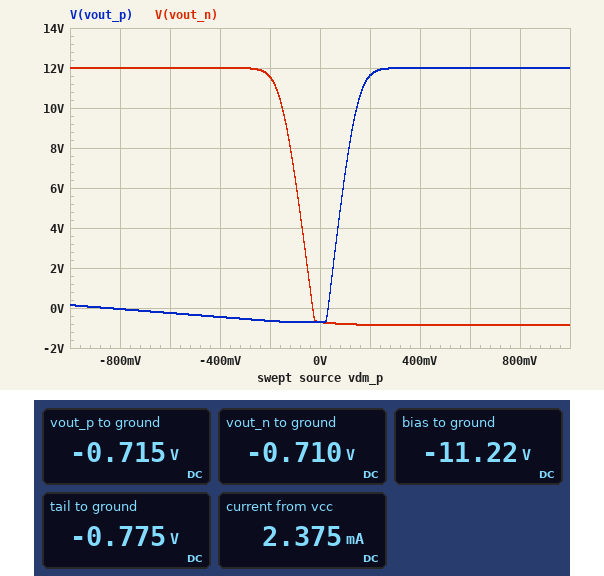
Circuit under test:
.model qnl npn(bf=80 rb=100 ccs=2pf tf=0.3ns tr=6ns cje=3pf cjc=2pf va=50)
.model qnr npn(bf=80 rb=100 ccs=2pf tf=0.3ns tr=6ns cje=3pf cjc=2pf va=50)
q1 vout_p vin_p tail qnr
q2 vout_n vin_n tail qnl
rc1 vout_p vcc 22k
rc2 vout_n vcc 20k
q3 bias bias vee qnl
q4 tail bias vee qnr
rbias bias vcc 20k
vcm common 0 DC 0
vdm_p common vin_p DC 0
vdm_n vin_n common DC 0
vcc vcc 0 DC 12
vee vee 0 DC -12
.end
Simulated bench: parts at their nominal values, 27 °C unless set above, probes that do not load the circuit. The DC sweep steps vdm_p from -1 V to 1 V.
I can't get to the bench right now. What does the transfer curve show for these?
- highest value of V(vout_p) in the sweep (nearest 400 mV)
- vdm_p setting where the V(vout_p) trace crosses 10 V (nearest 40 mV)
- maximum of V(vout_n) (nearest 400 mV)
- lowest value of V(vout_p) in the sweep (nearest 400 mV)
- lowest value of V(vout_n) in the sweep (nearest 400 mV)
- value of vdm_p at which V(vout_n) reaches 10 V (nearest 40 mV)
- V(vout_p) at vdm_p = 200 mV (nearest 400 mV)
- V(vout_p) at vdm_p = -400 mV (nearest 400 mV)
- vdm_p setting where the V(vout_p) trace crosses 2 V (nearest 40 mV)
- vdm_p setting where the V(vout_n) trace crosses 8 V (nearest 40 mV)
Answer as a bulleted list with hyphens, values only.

- 12.0 V
- 160 mV
- 12.0 V
- -800 mV
- -800 mV
- -160 mV
- 11.6 V
- -400 mV
- 40 mV
- -120 mV
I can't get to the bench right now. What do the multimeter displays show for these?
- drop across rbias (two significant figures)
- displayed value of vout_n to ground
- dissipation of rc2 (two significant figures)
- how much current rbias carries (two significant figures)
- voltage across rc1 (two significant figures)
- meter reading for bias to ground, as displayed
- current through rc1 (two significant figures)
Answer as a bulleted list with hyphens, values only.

- 23 V
- -0.710 V
- 8.1 mW
- 1.2 mA
- 13 V
- -11.22 V
- 580 µA
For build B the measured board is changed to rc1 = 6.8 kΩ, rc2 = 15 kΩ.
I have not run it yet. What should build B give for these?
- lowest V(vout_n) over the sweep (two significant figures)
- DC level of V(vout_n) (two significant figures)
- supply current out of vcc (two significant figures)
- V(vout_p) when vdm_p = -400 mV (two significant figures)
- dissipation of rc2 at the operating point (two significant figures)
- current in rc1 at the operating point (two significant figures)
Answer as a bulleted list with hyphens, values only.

- -810 mV
- 2.3 V
- 2.5 mA
- 2.7 V
- 6.3 mW
- 710 µA
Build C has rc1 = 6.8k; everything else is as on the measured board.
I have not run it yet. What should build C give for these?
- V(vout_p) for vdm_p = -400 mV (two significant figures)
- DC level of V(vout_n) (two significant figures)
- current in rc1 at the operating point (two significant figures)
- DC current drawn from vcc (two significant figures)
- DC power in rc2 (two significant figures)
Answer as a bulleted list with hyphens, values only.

- 2.7 V
- -560 mV
- 730 µA
- 2.5 mA
- 7.9 mW
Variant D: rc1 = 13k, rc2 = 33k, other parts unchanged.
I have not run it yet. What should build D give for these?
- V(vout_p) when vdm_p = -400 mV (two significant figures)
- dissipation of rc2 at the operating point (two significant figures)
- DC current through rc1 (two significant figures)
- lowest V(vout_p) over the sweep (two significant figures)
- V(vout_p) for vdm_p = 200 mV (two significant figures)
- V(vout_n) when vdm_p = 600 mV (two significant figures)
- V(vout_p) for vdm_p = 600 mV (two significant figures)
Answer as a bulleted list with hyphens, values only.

- -390 mV
- 4.9 mW
- 870 µA
- -680 mV
- 11 V
- -870 mV
- 12 V
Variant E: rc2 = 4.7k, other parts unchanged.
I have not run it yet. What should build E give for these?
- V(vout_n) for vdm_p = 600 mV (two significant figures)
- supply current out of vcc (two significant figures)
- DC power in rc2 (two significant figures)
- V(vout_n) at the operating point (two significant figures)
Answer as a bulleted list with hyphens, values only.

- 5.6 V
- 2.5 mA
- 2.7 mW
- 8.4 V
